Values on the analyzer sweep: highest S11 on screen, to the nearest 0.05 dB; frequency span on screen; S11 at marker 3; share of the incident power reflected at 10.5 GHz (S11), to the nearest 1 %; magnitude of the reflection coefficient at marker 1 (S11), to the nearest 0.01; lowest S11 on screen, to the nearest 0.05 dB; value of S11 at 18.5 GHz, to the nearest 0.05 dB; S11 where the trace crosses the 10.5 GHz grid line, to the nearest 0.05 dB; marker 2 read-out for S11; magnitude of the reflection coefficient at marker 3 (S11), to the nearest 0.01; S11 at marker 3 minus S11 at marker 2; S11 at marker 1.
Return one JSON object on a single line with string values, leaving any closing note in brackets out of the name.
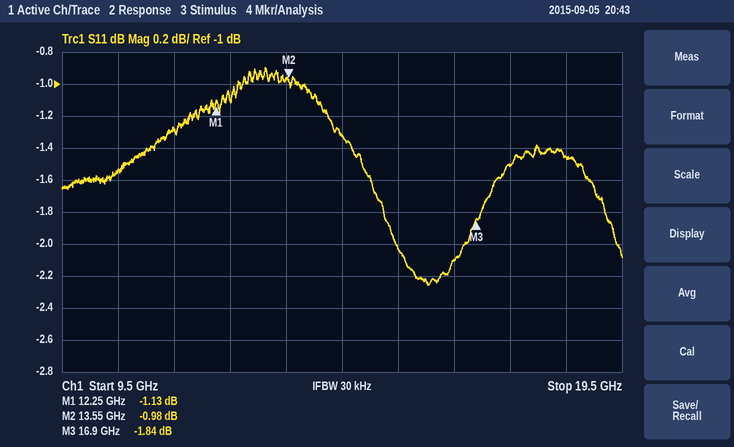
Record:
{"highest S11 on screen, to the nearest 0.05 dB": "-0.90 dB", "frequency span on screen": "10 GHz", "S11 at marker 3": "-1.84 dB", "share of the incident power reflected at 10.5 GHz (S11), to the nearest 1 %": "70 %", "magnitude of the reflection coefficient at marker 1 (S11), to the nearest 0.01": "0.88", "lowest S11 on screen, to the nearest 0.05 dB": "-2.25 dB", "value of S11 at 18.5 GHz, to the nearest 0.05 dB": "-1.45 dB", "S11 where the trace crosses the 10.5 GHz grid line, to the nearest 0.05 dB": "-1.55 dB", "marker 2 read-out for S11": "-0.98 dB", "magnitude of the reflection coefficient at marker 3 (S11), to the nearest 0.01": "0.81", "S11 at marker 3 minus S11 at marker 2": "-0.86 dB", "S11 at marker 1": "-1.13 dB"}
